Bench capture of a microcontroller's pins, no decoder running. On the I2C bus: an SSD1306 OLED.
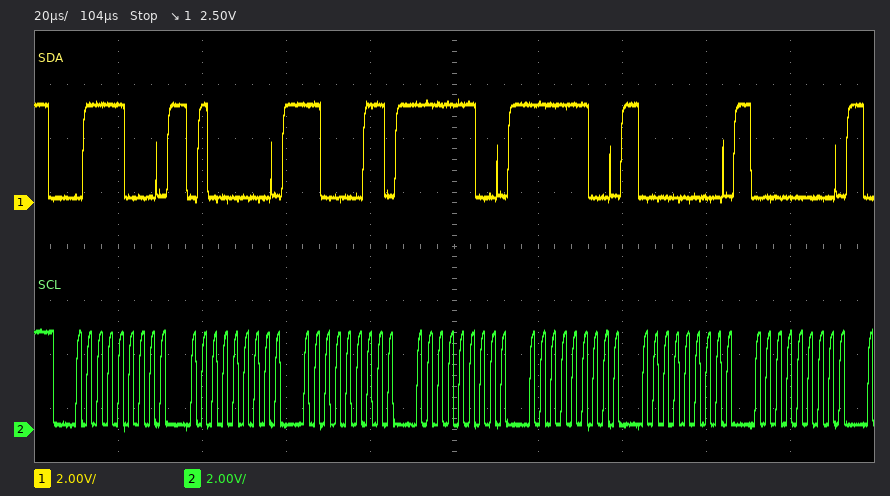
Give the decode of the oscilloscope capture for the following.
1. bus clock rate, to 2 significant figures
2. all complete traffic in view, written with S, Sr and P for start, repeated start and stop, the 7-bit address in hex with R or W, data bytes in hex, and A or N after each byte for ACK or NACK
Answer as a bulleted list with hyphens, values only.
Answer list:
- 400 kHz
- S 3CW A 40 A C3 A FC A FC A 00 A 00 A
